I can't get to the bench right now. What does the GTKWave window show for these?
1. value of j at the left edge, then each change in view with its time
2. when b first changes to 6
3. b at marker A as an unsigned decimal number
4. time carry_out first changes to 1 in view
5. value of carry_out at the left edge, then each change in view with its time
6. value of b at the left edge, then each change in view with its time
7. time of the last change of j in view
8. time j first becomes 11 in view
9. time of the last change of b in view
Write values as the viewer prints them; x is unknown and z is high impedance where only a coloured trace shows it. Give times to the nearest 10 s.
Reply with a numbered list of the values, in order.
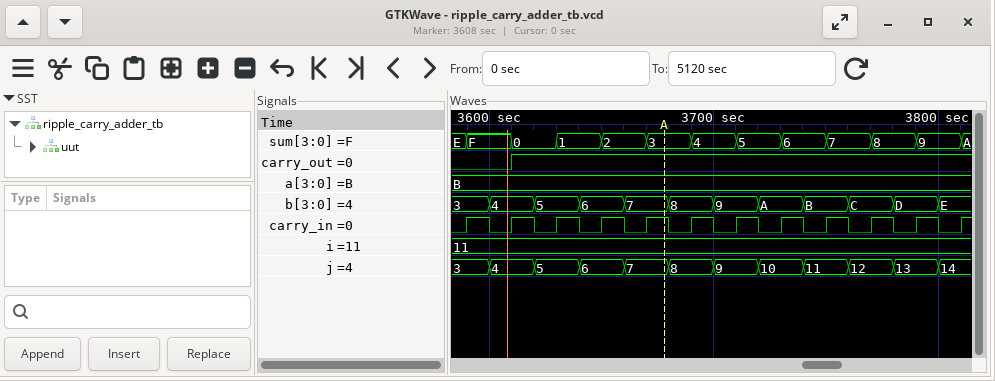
1. 3, 4 at 3600 s, 5 at 3620 s, 6 at 3640 s, 7 at 3660 s, 8 at 3680 s, 9 at 3700 s, 10 at 3720 s, 11 at 3740 s, 12 at 3760 s, 13 at 3780 s, 14 at 3800 s
2. 3640 s
3. 7
4. 3610 s
5. 0, 1 at 3610 s
6. 3, 4 at 3600 s, 5 at 3620 s, 6 at 3640 s, 7 at 3660 s, 8 at 3680 s, 9 at 3700 s, A at 3720 s, B at 3740 s, C at 3760 s, D at 3780 s, E at 3800 s
7. 3800 s
8. 3740 s
9. 3800 s
